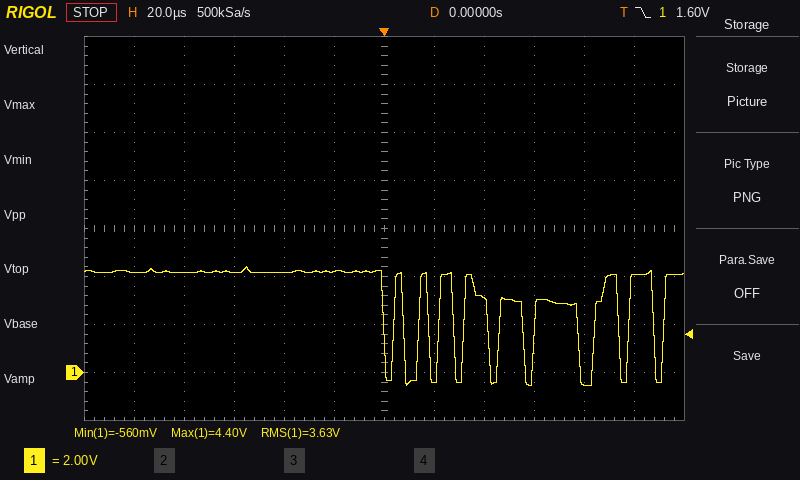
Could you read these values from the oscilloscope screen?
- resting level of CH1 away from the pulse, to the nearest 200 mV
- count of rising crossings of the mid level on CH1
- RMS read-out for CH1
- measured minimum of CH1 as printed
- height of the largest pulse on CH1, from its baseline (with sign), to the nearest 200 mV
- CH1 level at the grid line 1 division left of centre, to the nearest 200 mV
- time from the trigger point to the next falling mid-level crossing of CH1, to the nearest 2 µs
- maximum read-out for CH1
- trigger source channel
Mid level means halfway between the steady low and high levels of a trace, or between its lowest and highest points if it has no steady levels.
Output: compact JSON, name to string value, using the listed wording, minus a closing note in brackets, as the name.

{"resting level of CH1 away from the pulse, to the nearest 200 mV": "4.2 V", "count of rising crossings of the mid level on CH1": "9", "RMS read-out for CH1": "3.63 V", "measured minimum of CH1 as printed": "-560 mV", "height of the largest pulse on CH1, from its baseline (with sign), to the nearest 200 mV": "-4.8 V", "CH1 level at the grid line 1 division left of centre, to the nearest 200 mV": "4.2 V", "time from the trigger point to the next falling mid-level crossing of CH1, to the nearest 2 µs": "8 µs", "maximum read-out for CH1": "4.40 V", "trigger source channel": "CH1"}
